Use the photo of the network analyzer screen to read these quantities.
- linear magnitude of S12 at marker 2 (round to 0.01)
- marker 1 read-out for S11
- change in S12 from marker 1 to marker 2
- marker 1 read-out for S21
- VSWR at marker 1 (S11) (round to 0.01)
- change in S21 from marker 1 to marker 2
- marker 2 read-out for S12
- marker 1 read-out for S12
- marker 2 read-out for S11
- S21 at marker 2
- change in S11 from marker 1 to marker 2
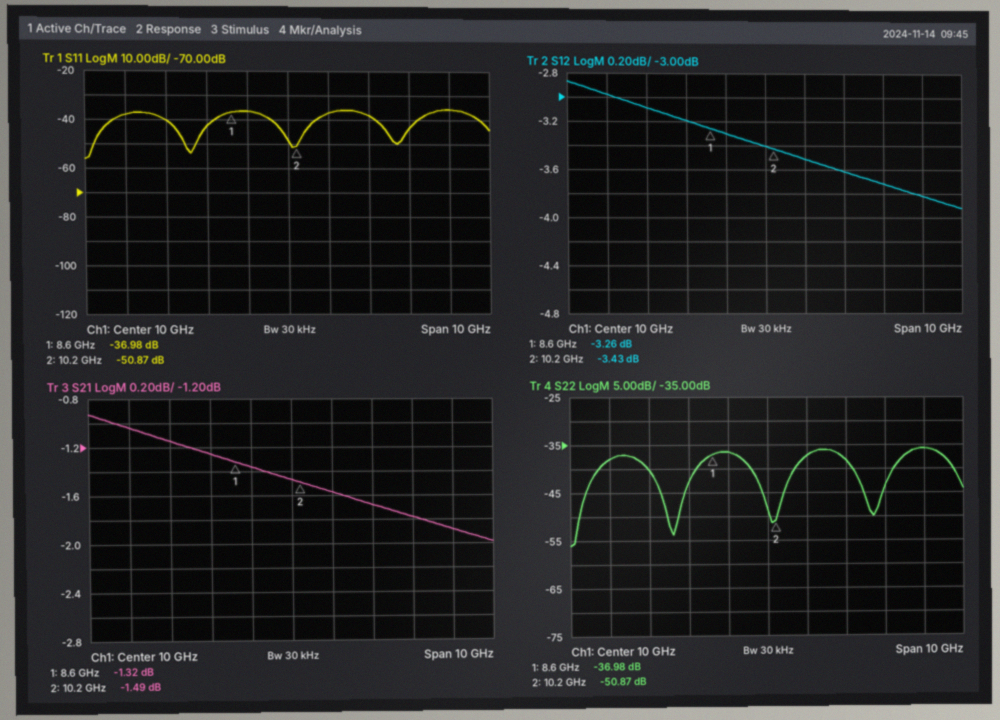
0.67
-36.98 dB
-0.17 dB
-1.32 dB
1.03
-0.17 dB
-3.43 dB
-3.26 dB
-50.87 dB
-1.49 dB
-13.89 dB
